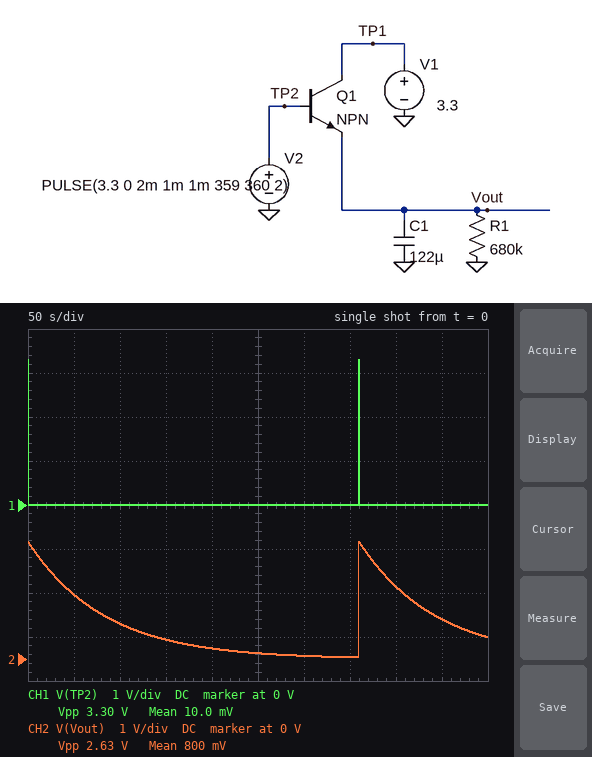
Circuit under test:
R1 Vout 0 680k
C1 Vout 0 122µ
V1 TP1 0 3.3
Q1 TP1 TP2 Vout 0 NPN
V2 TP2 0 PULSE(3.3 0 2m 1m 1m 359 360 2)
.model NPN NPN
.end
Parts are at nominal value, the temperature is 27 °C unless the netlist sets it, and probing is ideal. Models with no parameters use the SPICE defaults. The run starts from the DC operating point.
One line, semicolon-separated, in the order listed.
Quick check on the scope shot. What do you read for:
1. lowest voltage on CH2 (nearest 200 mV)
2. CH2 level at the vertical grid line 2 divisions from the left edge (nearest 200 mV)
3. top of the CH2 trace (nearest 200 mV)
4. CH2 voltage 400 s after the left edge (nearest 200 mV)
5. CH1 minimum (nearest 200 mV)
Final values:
0 V; 800 mV; 2.6 V; 1.6 V; 0 V
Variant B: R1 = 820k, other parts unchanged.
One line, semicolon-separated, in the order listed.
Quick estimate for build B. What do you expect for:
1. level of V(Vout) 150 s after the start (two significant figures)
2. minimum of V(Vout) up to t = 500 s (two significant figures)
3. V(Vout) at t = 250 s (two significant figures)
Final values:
600 mV; 74 mV; 220 mV
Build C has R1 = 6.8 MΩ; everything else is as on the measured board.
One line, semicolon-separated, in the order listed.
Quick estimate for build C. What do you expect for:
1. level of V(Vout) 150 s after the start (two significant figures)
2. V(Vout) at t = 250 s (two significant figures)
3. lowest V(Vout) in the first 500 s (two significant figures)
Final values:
2.3 V; 2.0 V; 1.8 V
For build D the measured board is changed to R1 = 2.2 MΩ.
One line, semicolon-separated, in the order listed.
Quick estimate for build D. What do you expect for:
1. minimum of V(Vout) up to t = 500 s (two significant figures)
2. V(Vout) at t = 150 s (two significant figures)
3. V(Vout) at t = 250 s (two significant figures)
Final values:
710 mV; 1.5 V; 1.1 V
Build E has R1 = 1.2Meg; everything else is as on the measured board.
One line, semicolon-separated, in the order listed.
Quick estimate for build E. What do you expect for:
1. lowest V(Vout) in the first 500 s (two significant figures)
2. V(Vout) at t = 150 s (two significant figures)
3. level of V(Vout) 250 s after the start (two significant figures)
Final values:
230 mV; 960 mV; 490 mV
